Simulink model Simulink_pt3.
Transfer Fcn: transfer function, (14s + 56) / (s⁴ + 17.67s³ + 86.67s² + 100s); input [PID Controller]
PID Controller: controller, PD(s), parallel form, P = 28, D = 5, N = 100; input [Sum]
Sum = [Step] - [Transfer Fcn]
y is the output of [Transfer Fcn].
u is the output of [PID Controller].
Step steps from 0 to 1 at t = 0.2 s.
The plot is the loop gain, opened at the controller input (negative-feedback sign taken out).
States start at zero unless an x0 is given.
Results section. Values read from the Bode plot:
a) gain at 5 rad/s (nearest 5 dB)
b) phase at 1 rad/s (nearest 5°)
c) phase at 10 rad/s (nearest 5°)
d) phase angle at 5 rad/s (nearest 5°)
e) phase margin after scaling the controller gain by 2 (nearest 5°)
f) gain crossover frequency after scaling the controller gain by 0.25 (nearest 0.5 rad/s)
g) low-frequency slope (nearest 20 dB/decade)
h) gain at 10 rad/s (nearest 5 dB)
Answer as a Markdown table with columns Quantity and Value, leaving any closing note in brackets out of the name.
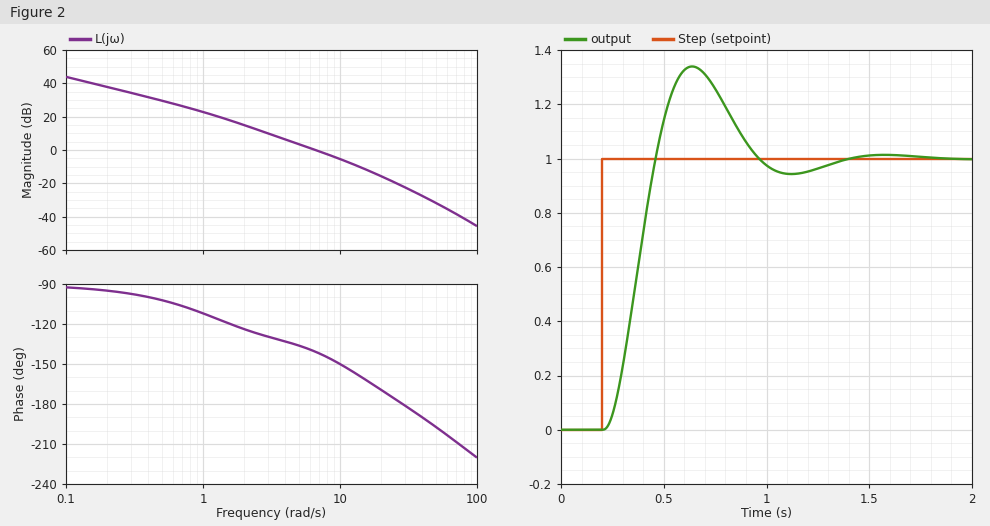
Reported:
| Quantity | Value |
|---|---|
| gain at 5 rad/s | 5 dB |
| phase at 1 rad/s | -110° |
| phase at 10 rad/s | -150° |
| phase angle at 5 rad/s | -135° |
| phase margin after scaling the controller gain by 2 | 30° |
| gain crossover frequency after scaling the controller gain by 0.25 | 2.5 rad/s |
| low-frequency slope | -20 dB/decade |
| gain at 10 rad/s | -5 dB |
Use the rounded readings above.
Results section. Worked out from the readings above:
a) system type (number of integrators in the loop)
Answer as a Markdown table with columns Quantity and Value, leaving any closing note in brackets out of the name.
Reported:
| Quantity | Value |
|---|---|
| system type | 1 |
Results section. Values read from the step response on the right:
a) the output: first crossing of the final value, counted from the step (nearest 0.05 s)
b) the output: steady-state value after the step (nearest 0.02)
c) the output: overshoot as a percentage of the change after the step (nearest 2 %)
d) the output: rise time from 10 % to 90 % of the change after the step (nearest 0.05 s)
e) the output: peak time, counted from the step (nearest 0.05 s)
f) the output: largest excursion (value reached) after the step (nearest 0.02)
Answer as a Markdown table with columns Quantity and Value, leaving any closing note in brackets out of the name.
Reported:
| Quantity | Value |
|---|---|
| the output: first crossing of the final value, counted from the step | 0.25 s |
| the output: steady-state value after the step | 1.00 |
| the output: overshoot as a percentage of the change after the step | 34 % |
| the output: rise time from 10 % to 90 % of the change after the step | 0.15 s |
| the output: peak time, counted from the step | 0.45 s |
| the output: largest excursion (value reached) after the step | 1.34 |
